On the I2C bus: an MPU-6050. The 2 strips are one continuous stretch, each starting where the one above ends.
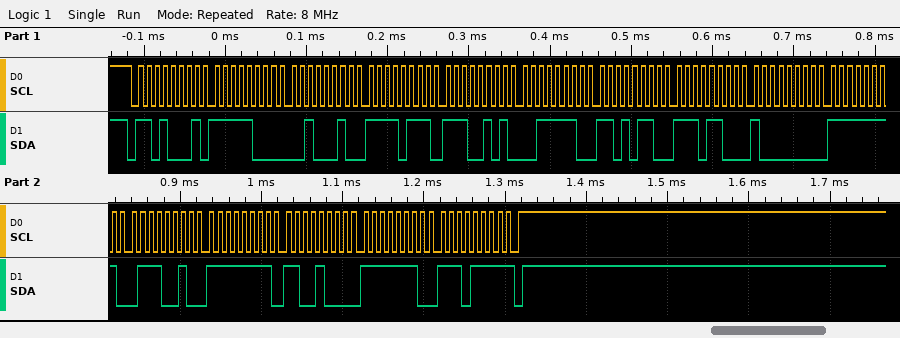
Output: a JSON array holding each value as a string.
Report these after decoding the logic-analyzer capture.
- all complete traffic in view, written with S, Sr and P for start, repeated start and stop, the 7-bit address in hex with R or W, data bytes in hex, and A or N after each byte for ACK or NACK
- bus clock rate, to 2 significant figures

["S 68R A F8 A 22 A F7 A E5 A 3E A D6 A EC A 80 A FF A 72 A FF A C8 A FE A EF N P", "100 kHz"]
